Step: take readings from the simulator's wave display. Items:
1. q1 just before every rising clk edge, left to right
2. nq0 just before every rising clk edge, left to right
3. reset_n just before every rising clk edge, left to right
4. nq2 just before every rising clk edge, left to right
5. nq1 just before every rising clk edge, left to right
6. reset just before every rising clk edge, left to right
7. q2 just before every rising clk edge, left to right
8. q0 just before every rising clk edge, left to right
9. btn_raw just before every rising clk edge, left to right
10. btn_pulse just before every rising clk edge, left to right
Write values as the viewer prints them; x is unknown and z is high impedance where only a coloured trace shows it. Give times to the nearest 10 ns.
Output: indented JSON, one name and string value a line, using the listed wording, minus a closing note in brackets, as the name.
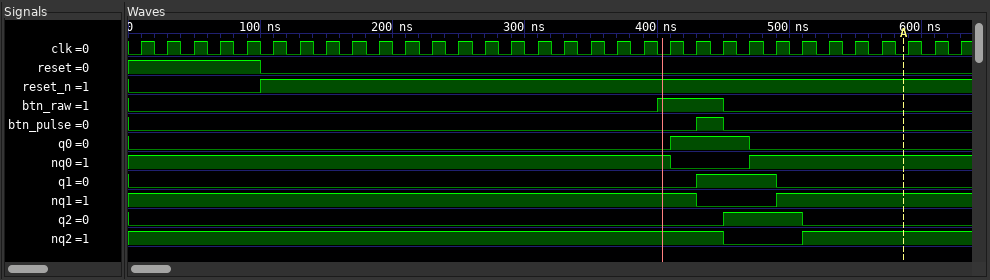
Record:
{
  "q1 just before every rising clk edge, left to right": "0 0 0 0 0 0 0 0 0 0 0 0 0 0 0 0 0 0 0 0 0 0 1 1 1 0 0 0 0 0 0 0",
  "nq0 just before every rising clk edge, left to right": "1 1 1 1 1 1 1 1 1 1 1 1 1 1 1 1 1 1 1 1 1 0 0 0 1 1 1 1 1 1 1 1",
  "reset_n just before every rising clk edge, left to right": "0 0 0 0 0 1 1 1 1 1 1 1 1 1 1 1 1 1 1 1 1 1 1 1 1 1 1 1 1 1 1 1",
  "nq2 just before every rising clk edge, left to right": "1 1 1 1 1 1 1 1 1 1 1 1 1 1 1 1 1 1 1 1 1 1 1 0 0 0 1 1 1 1 1 1",
  "nq1 just before every rising clk edge, left to right": "1 1 1 1 1 1 1 1 1 1 1 1 1 1 1 1 1 1 1 1 1 1 0 0 0 1 1 1 1 1 1 1",
  "reset just before every rising clk edge, left to right": "1 1 1 1 1 0 0 0 0 0 0 0 0 0 0 0 0 0 0 0 0 0 0 0 0 0 0 0 0 0 0 0",
  "q2 just before every rising clk edge, left to right": "0 0 0 0 0 0 0 0 0 0 0 0 0 0 0 0 0 0 0 0 0 0 0 1 1 1 0 0 0 0 0 0",
  "q0 just before every rising clk edge, left to right": "0 0 0 0 0 0 0 0 0 0 0 0 0 0 0 0 0 0 0 0 0 1 1 1 0 0 0 0 0 0 0 0",
  "btn_raw just before every rising clk edge, left to right": "0 0 0 0 0 0 0 0 0 0 0 0 0 0 0 0 0 0 0 0 1 1 1 0 0 0 0 0 0 0 0 0",
  "btn_pulse just before every rising clk edge, left to right": "0 0 0 0 0 0 0 0 0 0 0 0 0 0 0 0 0 0 0 0 0 0 1 0 0 0 0 0 0 0 0 0"
}
